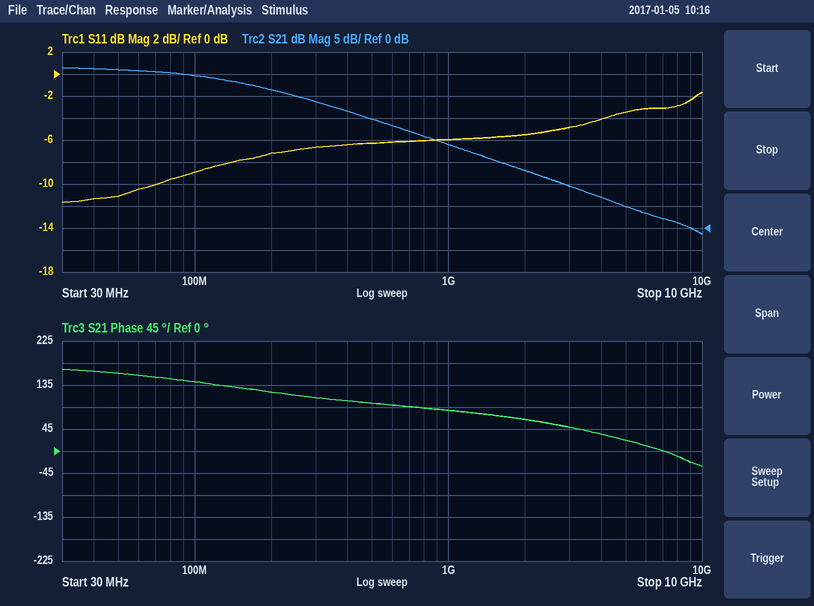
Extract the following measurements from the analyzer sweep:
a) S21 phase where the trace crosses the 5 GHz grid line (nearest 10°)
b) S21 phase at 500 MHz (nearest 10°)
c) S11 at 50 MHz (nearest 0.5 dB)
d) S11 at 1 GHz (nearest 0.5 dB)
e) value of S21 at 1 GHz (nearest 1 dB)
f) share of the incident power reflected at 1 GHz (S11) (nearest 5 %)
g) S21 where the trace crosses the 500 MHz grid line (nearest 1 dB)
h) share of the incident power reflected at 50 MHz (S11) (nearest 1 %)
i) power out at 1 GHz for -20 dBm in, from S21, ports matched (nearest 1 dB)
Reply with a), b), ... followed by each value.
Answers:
a) 20°
b) 100°
c) -11.0 dB
d) -6.0 dB
e) 19 dB
f) 25 %
g) 25 dB
h) 8 %
i) -1 dBm
